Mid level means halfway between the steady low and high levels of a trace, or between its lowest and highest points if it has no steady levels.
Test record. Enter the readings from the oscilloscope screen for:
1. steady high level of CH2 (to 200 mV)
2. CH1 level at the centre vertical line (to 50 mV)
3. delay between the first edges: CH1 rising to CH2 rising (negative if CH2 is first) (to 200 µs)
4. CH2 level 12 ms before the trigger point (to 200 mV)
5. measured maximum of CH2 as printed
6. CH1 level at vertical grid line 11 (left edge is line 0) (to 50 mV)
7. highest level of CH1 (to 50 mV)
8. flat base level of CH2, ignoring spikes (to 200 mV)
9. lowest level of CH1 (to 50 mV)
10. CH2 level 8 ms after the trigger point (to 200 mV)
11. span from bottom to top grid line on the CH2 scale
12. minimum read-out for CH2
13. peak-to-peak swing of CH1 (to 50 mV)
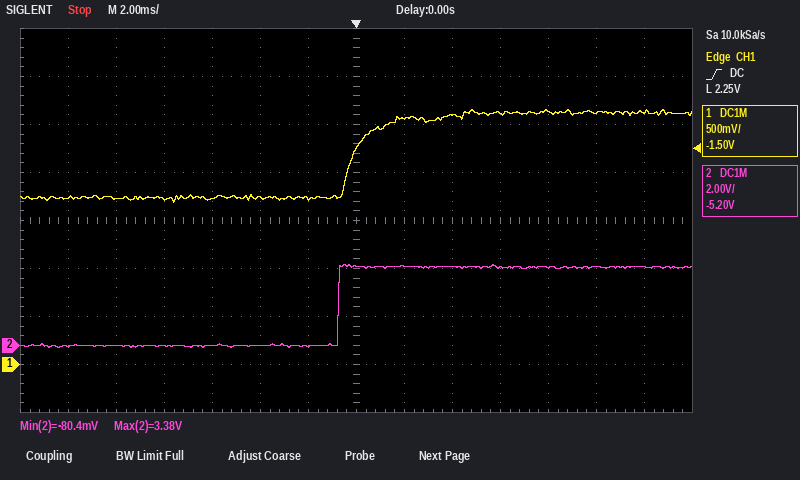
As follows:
3.2 V
2.25 V
-600 µs
0.0 V
3.38 V
2.65 V
2.65 V
0.0 V
1.70 V
3.2 V
16 V
-80.4 mV
950 mV
